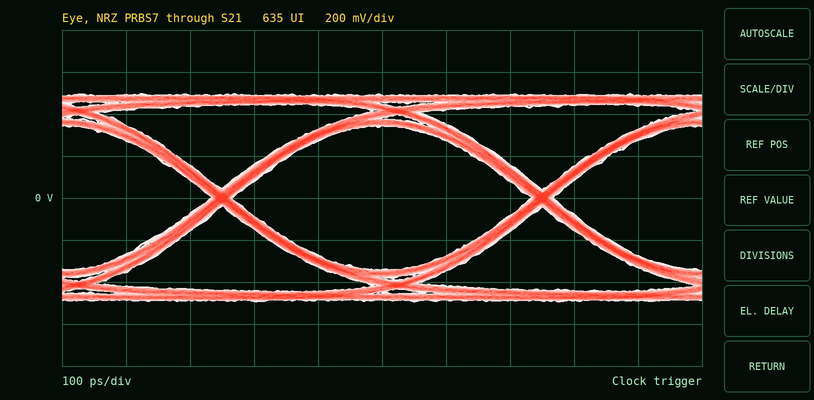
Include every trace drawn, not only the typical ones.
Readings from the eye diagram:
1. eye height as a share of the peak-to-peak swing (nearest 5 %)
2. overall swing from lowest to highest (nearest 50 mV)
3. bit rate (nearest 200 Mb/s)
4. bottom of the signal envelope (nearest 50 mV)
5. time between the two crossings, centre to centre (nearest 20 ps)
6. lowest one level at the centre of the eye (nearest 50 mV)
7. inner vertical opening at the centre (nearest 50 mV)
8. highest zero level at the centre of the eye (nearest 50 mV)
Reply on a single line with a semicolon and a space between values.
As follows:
70 %; 1.00 V; 2.0 Gb/s; -500 mV; 500 ps; 350 mV; 700 mV; -350 mV
